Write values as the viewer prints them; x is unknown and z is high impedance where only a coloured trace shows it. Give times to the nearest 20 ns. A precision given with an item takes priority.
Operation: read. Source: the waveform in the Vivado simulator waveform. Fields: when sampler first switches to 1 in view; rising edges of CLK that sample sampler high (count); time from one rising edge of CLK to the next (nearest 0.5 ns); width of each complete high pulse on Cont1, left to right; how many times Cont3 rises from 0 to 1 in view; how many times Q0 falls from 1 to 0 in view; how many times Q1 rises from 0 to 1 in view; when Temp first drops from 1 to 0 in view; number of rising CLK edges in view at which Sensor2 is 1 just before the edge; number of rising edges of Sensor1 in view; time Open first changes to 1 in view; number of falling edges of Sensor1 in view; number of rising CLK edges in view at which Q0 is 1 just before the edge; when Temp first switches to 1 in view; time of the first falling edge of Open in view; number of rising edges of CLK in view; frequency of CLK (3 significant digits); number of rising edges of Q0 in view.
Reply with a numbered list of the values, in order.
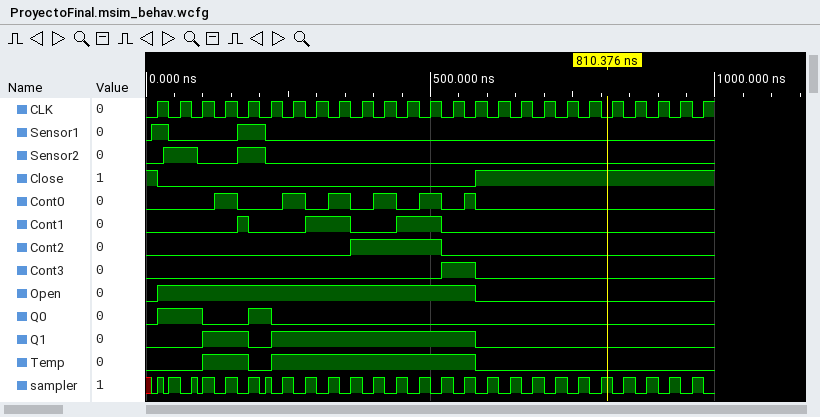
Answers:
1. 20 ns
2. 21
3. 40 ns
4. 20 ns, 80 ns, 80 ns
5. 1
6. 2
7. 2
8. 180 ns
9. 2
10. 2
11. 20 ns
12. 2
13. 3
14. 100 ns
15. 580 ns
16. 25
17. 25.0 MHz
18. 2
